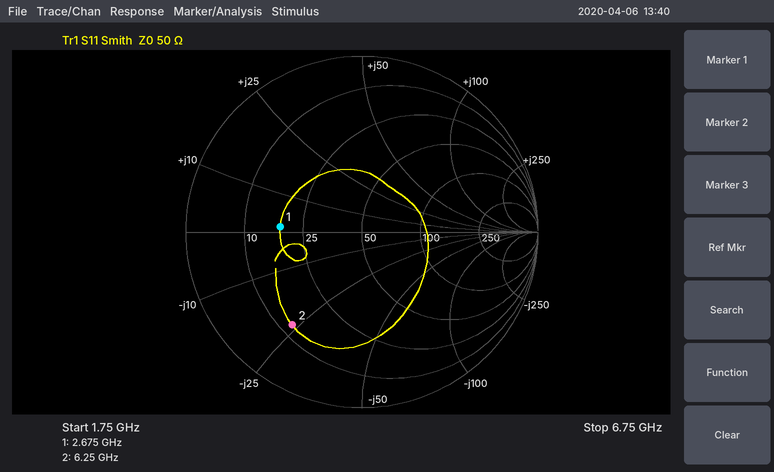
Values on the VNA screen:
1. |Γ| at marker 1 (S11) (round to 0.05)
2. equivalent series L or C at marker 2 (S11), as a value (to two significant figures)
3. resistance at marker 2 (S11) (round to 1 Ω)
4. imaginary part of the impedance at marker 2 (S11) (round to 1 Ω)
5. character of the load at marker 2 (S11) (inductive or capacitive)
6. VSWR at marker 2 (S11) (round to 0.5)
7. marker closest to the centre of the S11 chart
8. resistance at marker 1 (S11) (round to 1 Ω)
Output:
0.45
1.1 pF
13 Ω
-24 Ω
capacitive
5.0
marker 1
18 Ω
